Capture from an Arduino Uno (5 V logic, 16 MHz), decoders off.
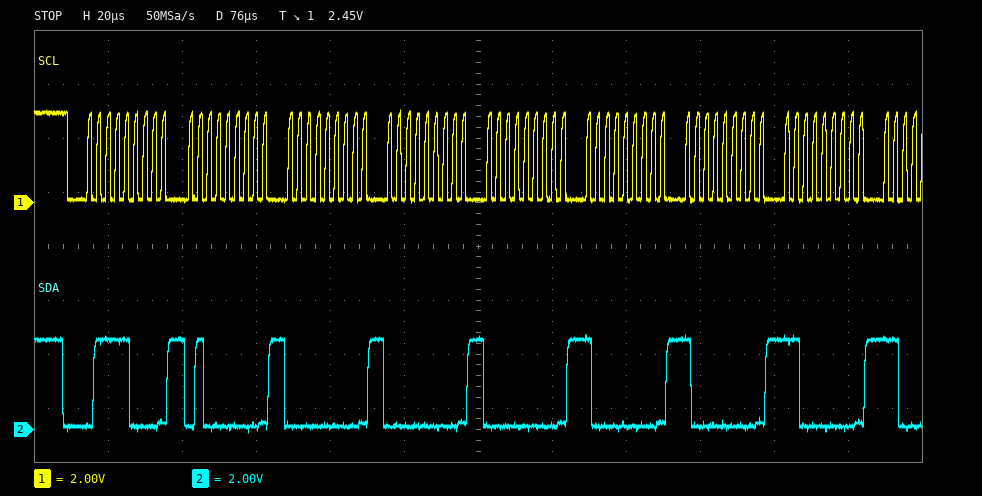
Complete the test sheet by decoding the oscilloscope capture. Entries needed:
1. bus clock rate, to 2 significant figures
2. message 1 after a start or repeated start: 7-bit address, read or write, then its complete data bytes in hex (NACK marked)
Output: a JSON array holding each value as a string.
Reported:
["400 kHz", "0x3C write: 40 00 00 00 80 80 C0"]
